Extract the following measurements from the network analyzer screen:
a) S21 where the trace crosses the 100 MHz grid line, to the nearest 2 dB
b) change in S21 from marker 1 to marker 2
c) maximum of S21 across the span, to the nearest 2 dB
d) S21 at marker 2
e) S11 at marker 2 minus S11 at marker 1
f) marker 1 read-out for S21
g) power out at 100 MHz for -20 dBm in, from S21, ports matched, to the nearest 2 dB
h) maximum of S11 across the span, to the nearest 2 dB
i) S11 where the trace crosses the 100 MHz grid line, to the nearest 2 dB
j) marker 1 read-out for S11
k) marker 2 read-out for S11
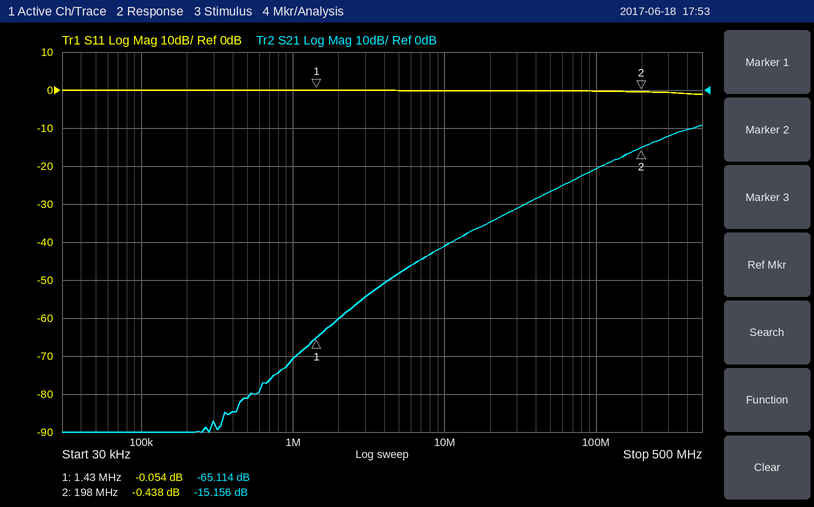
-20 dB
49.958 dB
-10 dB
-15.156 dB
-0.384 dB
-65.114 dB
-40 dBm
0 dB
0 dB
-0.054 dB
-0.438 dB
